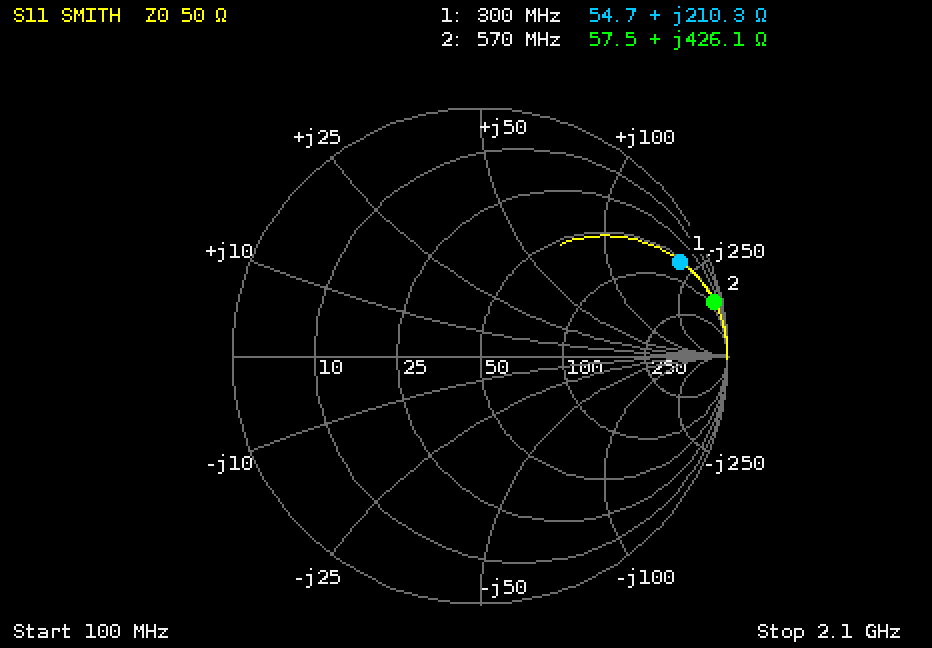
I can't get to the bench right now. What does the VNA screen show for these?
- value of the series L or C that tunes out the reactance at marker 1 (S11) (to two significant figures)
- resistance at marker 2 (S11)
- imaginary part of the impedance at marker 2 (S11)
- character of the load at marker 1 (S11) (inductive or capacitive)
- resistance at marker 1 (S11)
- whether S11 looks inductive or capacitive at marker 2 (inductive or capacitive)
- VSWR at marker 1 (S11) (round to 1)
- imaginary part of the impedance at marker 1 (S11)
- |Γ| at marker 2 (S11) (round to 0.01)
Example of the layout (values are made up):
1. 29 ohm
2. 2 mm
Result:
1. 2.5 pF
2. 57.5 Ω
3. +426.1 Ω
4. inductive
5. 54.7 Ω
6. inductive
7. 18
8. +210.3 Ω
9. 0.97
